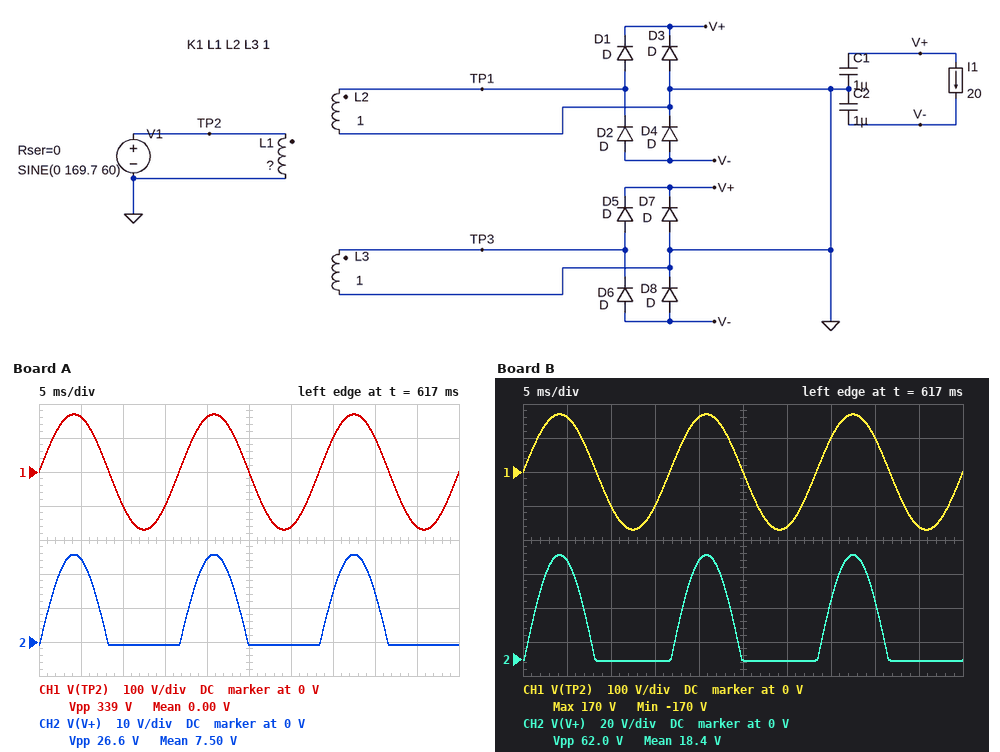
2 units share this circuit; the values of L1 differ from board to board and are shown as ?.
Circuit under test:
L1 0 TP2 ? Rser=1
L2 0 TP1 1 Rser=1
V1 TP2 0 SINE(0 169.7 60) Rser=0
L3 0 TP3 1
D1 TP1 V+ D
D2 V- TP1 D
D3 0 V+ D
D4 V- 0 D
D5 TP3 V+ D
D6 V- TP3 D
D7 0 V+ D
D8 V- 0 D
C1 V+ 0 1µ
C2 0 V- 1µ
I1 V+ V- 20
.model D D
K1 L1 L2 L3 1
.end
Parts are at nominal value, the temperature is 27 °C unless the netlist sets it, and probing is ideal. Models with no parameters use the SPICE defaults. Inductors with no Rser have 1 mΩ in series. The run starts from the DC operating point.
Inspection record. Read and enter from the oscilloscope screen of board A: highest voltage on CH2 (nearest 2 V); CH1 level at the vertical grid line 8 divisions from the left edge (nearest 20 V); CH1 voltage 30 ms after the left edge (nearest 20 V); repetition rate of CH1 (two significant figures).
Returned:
26 V
100 V
-160 V
60 Hz
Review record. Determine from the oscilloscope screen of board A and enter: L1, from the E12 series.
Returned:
39 H
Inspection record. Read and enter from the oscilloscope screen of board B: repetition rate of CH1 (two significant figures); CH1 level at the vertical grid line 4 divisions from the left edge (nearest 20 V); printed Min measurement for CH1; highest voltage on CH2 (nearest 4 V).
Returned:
60 Hz
160 V
-170 V
60 V
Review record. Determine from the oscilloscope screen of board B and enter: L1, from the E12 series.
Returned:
6.8 H
